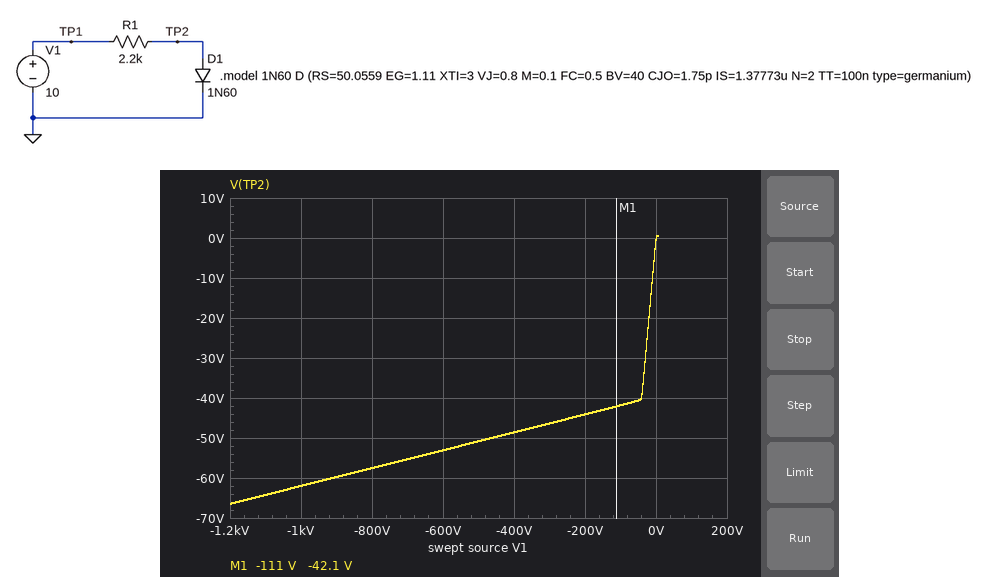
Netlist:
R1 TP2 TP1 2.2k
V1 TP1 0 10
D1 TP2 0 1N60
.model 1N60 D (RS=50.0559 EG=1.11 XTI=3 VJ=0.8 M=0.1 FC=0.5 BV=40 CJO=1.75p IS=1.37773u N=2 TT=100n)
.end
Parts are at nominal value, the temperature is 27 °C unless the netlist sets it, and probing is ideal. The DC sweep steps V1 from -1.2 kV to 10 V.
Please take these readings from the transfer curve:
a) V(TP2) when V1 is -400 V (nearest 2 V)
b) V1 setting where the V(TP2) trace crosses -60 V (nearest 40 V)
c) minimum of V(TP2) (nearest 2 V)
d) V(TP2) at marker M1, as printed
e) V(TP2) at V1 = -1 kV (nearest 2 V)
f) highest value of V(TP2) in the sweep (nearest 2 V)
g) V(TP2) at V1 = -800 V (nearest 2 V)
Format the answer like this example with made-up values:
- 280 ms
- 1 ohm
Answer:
- -48 V
- -920 V
- -66 V
- -42.1 V
- -62 V
- 0 V
- -58 V
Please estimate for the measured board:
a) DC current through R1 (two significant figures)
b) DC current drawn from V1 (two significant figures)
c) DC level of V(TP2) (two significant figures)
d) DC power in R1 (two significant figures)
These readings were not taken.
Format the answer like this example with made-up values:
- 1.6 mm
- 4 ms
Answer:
- 4.3 mA
- 4.3 mA
- 630 mV
- 40 mW
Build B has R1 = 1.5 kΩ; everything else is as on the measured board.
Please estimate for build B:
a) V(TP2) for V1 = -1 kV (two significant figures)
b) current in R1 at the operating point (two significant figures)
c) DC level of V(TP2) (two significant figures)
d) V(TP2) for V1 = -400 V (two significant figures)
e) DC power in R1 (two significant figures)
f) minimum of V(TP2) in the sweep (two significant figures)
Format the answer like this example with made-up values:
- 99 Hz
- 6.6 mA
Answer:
- -72 V
- 6.2 mA
- 740 mV
- -52 V
- 57 mW
- -78 V
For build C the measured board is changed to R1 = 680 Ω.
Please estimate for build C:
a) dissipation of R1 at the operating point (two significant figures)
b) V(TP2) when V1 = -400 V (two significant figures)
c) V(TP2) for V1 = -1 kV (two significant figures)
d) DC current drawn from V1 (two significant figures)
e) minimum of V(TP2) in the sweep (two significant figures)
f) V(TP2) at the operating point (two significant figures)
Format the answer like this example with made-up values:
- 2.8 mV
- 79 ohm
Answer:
- 120 mW
- -65 V
- -110 V
- 13 mA
- -120 V
- 1.1 V
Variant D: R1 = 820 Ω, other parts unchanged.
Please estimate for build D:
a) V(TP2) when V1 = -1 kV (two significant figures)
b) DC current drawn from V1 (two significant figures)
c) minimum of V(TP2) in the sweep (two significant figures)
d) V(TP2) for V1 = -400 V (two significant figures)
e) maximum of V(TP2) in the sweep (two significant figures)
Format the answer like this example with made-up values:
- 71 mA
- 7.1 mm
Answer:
- -96 V
- 11 mA
- -110 V
- -61 V
- 1.0 V
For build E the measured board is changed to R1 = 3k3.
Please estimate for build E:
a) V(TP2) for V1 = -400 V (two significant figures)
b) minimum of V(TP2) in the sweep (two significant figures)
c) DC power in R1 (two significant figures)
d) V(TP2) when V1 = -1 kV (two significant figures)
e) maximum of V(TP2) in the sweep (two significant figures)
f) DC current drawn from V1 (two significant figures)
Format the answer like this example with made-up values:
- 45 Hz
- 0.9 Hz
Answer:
- -46 V
- -58 V
- 27 mW
- -55 V
- 540 mV
- 2.9 mA
